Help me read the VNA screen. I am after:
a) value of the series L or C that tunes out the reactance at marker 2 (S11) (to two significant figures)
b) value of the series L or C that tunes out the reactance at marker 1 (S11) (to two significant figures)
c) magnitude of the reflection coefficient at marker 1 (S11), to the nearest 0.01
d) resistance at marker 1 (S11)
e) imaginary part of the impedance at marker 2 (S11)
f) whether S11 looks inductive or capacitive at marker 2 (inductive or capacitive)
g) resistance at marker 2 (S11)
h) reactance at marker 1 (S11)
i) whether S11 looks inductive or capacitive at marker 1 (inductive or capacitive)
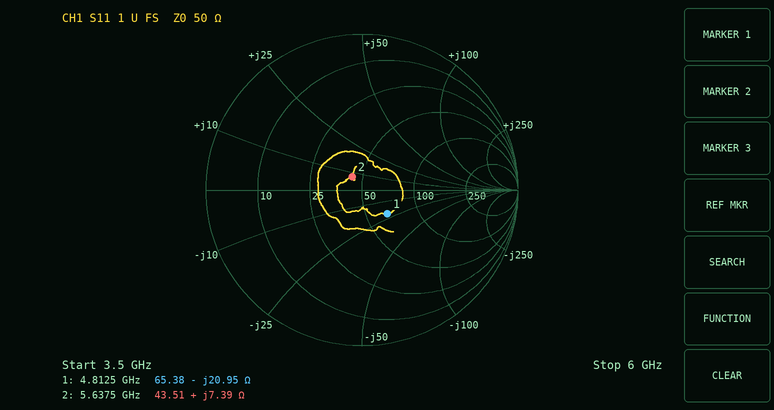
3.8 pF
690 pH
0.22
65.38 Ω
+7.39 Ω
inductive
43.51 Ω
-20.95 Ω
capacitive
